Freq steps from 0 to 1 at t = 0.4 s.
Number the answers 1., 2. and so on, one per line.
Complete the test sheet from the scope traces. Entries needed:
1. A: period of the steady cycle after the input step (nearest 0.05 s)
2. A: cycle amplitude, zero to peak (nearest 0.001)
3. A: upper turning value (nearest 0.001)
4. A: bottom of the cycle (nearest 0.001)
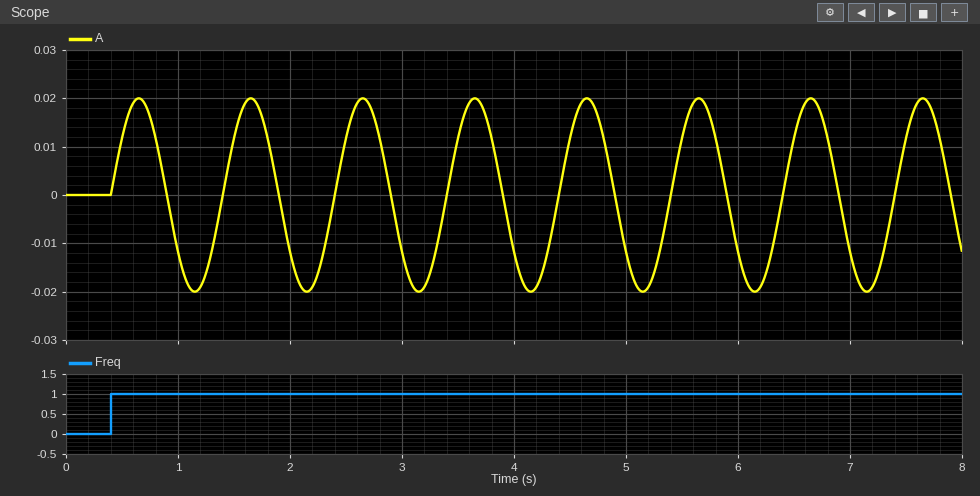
1. 1.00 s
2. 0.020
3. 0.020
4. -0.020
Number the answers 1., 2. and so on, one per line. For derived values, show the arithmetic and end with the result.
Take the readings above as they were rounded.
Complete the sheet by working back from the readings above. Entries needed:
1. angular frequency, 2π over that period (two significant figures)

1. 2π / 1 = 6.3 rad/s
